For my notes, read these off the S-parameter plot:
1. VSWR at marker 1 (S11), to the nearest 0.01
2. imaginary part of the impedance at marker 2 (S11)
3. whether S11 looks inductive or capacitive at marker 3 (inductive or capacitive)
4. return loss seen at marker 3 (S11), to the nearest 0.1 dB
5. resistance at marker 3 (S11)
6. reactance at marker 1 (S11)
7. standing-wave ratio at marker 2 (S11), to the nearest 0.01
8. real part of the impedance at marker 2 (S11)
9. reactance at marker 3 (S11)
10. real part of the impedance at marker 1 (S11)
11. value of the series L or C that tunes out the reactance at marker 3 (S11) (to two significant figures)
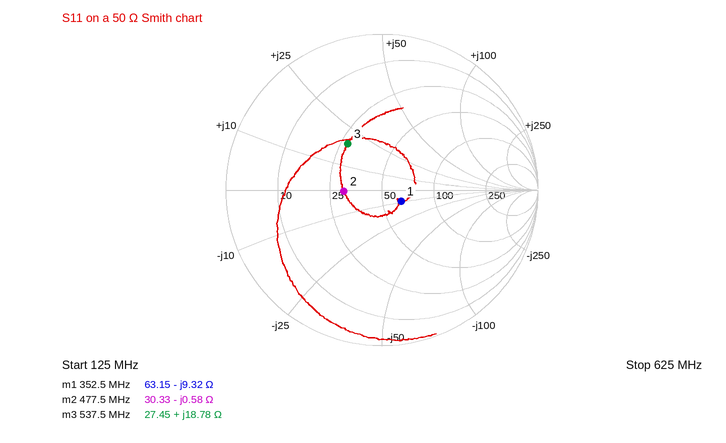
1.33
-0.58 Ω
inductive
8.7 dB
27.45 Ω
-9.32 Ω
1.65
30.33 Ω
+18.78 Ω
63.15 Ω
16 pF
